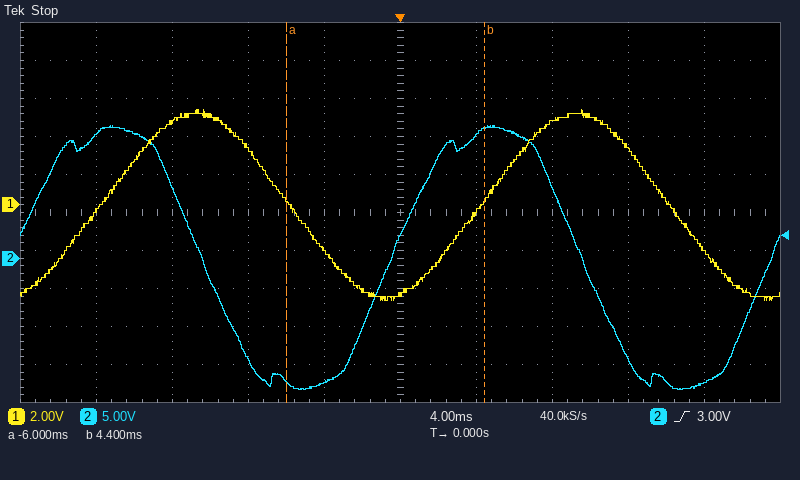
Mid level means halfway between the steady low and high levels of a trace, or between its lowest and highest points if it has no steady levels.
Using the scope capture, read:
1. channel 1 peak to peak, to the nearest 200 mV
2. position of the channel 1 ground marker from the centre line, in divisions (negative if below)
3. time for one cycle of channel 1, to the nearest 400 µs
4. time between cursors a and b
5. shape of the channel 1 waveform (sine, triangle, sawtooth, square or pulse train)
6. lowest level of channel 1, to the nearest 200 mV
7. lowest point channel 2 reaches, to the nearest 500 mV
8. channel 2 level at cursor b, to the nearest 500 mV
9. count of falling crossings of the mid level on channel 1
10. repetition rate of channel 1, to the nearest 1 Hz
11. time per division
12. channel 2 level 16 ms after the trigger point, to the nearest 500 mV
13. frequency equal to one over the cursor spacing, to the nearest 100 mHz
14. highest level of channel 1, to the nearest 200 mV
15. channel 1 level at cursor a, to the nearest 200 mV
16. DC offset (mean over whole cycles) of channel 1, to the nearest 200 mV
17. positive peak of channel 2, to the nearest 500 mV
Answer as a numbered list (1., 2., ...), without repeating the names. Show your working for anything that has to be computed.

1. 5.0 V − (-5.0 V) = 10.0 V
2. +0.2 div
3. 20.0 ms
4. 4.4 ms − (-6 ms) = 10.4 ms
5. sine
6. -5.0 V
7. -17.5 V
8. 17.0 V
9. 2
10. 1 / 20.0 ms ≈ 50 Hz
11. 4 ms
12. -16.5 V
13. 1 / 10.4 ms ≈ 96.2 Hz
14. 5.0 V
15. 200 mV
16. (5.0 V + (-5.0 V)) / 2 ≈ 0.0 V
17. 17.5 V
